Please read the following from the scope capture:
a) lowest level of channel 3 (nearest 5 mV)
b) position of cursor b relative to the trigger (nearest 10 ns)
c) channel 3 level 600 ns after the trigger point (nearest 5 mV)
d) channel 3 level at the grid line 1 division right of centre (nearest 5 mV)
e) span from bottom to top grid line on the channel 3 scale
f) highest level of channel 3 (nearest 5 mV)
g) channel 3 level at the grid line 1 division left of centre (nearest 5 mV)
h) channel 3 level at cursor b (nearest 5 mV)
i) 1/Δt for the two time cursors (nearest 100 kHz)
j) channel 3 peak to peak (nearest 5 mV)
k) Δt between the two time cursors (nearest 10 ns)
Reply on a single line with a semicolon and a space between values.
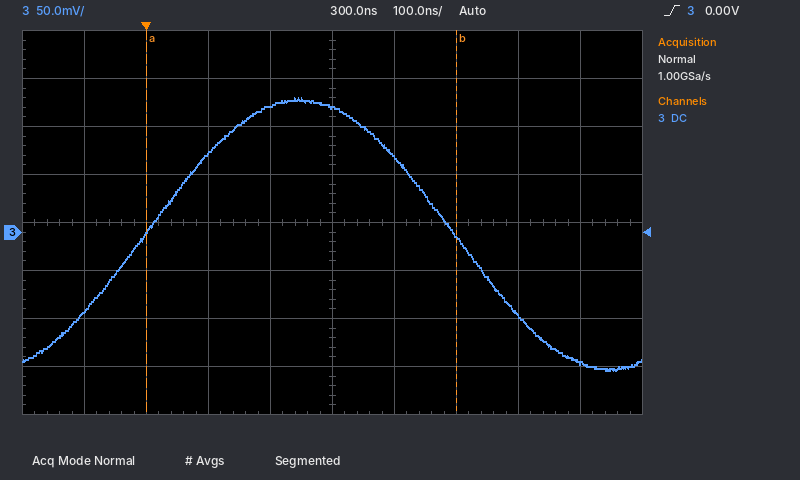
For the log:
-145 mV; +500 ns; -85 mV; 80 mV; 400 mV; 140 mV; 130 mV; -5 mV; 2.0 MHz; 285 mV; 500 ns
